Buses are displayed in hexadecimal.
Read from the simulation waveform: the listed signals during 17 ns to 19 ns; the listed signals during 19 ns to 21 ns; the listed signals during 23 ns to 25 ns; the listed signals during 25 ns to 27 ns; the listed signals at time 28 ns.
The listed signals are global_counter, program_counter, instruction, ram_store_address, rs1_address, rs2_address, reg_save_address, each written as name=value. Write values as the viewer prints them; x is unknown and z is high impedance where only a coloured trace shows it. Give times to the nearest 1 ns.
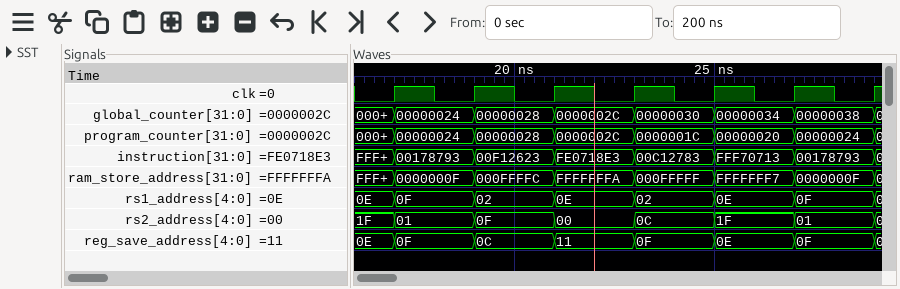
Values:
global_counter=00000024, program_counter=00000024, instruction=00178793, ram_store_address=0000000F, rs1_address=0F, rs2_address=01, reg_save_address=0F
global_counter=00000028, program_counter=00000028, instruction=00F12623, ram_store_address=000FFFFC, rs1_address=02, rs2_address=0F, reg_save_address=0C
global_counter=00000030, program_counter=0000001C, instruction=00C12783, ram_store_address=000FFFFF, rs1_address=02, rs2_address=0C, reg_save_address=0F
global_counter=00000034, program_counter=00000020, instruction=FFF70713, ram_store_address=FFFFFFF7, rs1_address=0E, rs2_address=1F, reg_save_address=0E
global_counter=00000038, program_counter=00000024, instruction=00178793, ram_store_address=0000000F, rs1_address=0F, rs2_address=01, reg_save_address=0F
